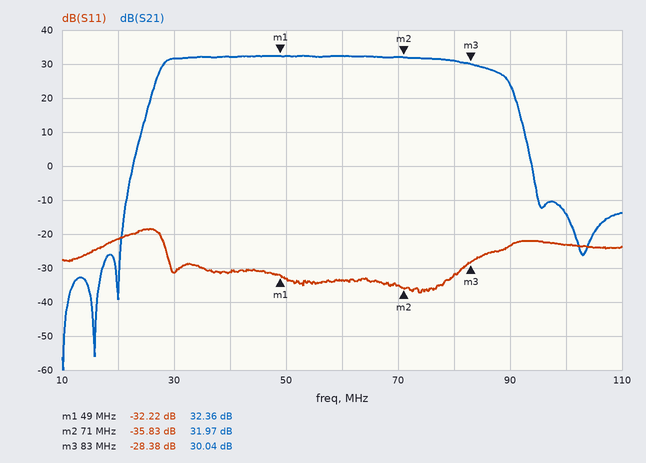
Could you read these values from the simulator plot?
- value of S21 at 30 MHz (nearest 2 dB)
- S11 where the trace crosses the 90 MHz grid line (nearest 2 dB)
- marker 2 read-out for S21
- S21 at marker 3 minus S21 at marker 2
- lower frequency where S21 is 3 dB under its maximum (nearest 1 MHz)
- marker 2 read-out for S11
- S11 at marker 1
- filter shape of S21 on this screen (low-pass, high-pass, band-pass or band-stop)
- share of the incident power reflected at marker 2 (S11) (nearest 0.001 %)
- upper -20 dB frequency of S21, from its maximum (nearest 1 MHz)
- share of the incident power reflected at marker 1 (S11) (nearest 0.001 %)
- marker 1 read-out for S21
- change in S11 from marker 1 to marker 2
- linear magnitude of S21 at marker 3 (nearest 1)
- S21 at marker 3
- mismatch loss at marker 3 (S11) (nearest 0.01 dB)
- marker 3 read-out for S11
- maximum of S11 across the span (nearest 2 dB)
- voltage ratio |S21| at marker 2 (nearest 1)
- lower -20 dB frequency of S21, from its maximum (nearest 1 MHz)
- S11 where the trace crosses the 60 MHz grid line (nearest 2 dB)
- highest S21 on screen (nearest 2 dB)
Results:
32 dB
-24 dB
31.97 dB
-1.93 dB
28 MHz
-35.83 dB
-32.22 dB
band-pass
0.026 %
92 MHz
0.060 %
32.36 dB
-3.61 dB
32
30.04 dB
0.01 dB
-28.38 dB
-18 dB
40
25 MHz
-34 dB
32 dB
